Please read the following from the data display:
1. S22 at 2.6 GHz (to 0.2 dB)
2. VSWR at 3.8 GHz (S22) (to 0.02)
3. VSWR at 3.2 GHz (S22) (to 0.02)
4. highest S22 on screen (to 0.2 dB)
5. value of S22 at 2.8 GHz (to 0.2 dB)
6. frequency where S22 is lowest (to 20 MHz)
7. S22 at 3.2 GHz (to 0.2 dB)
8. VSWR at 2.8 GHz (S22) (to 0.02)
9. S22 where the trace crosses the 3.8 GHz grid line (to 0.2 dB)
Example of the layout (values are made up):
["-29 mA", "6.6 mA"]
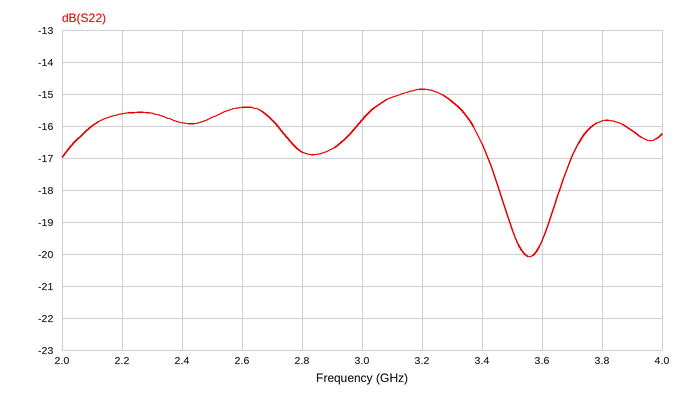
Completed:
["-15.4 dB", "1.38", "1.44", "-14.8 dB", "-16.8 dB", "3.56 GHz", "-14.8 dB", "1.34", "-15.8 dB"]
